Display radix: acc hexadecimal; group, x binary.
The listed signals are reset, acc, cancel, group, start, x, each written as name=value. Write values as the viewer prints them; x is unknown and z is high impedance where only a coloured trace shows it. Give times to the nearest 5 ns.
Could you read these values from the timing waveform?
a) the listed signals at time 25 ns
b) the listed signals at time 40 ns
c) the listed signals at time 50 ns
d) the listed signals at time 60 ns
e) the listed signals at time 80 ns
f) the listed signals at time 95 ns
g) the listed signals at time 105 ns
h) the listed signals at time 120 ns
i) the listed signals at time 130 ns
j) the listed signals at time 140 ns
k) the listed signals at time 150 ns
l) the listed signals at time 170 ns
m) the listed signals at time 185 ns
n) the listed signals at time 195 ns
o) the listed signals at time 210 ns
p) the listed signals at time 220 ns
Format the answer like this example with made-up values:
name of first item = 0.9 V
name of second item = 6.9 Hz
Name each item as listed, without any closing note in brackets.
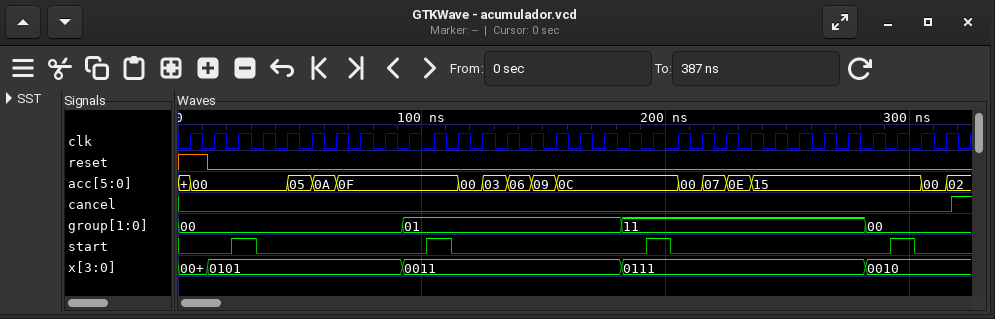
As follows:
the listed signals at time 25 ns = reset=0, acc=00, cancel=0, group=00, start=1, x=0101
the listed signals at time 40 ns = reset=0, acc=00, cancel=0, group=00, start=0, x=0101
the listed signals at time 50 ns = reset=0, acc=05, cancel=0, group=00, start=0, x=0101
the listed signals at time 60 ns = reset=0, acc=0A, cancel=0, group=00, start=0, x=0101
the listed signals at time 80 ns = reset=0, acc=0F, cancel=0, group=00, start=0, x=0101
the listed signals at time 95 ns = reset=0, acc=0F, cancel=0, group=01, start=0, x=0011
the listed signals at time 105 ns = reset=0, acc=0F, cancel=0, group=01, start=1, x=0011
the listed signals at time 120 ns = reset=0, acc=00, cancel=0, group=01, start=0, x=0011
the listed signals at time 130 ns = reset=0, acc=03, cancel=0, group=01, start=0, x=0011
the listed signals at time 140 ns = reset=0, acc=06, cancel=0, group=01, start=0, x=0011
the listed signals at time 150 ns = reset=0, acc=09, cancel=0, group=01, start=0, x=0011
the listed signals at time 170 ns = reset=0, acc=0C, cancel=0, group=01, start=0, x=0011
the listed signals at time 185 ns = reset=0, acc=0C, cancel=0, group=11, start=0, x=0111
the listed signals at time 195 ns = reset=0, acc=0C, cancel=0, group=11, start=1, x=0111
the listed signals at time 210 ns = reset=0, acc=00, cancel=0, group=11, start=0, x=0111
the listed signals at time 220 ns = reset=0, acc=07, cancel=0, group=11, start=0, x=0111
